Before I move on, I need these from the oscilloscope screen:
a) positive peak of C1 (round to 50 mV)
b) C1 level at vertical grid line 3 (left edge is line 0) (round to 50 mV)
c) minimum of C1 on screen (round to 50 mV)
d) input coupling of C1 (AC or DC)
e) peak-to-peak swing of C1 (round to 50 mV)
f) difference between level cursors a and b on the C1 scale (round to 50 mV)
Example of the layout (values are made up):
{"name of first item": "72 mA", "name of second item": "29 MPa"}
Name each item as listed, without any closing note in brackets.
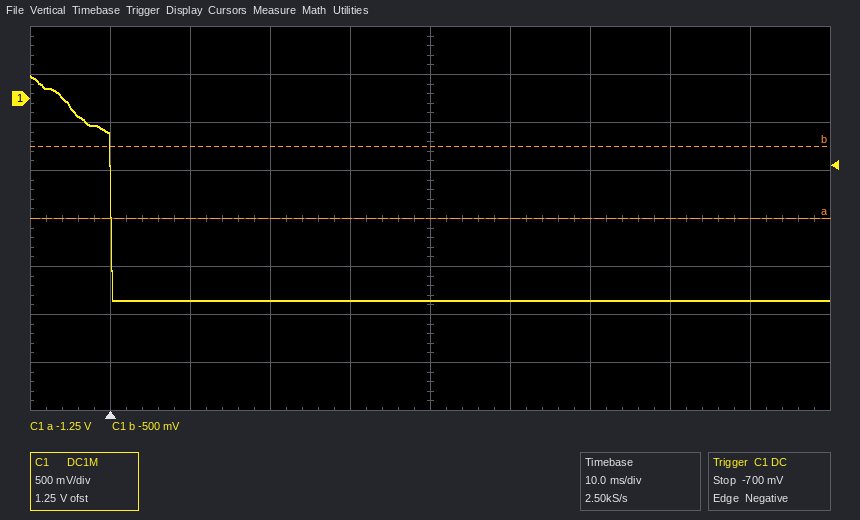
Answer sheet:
{"positive peak of C1": "250 mV", "C1 level at vertical grid line 3 (left edge is line 0)": "-2.10 V", "minimum of C1 on screen": "-2.10 V", "input coupling of C1": "DC", "peak-to-peak swing of C1": "2.35 V", "difference between level cursors a and b on the C1 scale": "750 mV"}
